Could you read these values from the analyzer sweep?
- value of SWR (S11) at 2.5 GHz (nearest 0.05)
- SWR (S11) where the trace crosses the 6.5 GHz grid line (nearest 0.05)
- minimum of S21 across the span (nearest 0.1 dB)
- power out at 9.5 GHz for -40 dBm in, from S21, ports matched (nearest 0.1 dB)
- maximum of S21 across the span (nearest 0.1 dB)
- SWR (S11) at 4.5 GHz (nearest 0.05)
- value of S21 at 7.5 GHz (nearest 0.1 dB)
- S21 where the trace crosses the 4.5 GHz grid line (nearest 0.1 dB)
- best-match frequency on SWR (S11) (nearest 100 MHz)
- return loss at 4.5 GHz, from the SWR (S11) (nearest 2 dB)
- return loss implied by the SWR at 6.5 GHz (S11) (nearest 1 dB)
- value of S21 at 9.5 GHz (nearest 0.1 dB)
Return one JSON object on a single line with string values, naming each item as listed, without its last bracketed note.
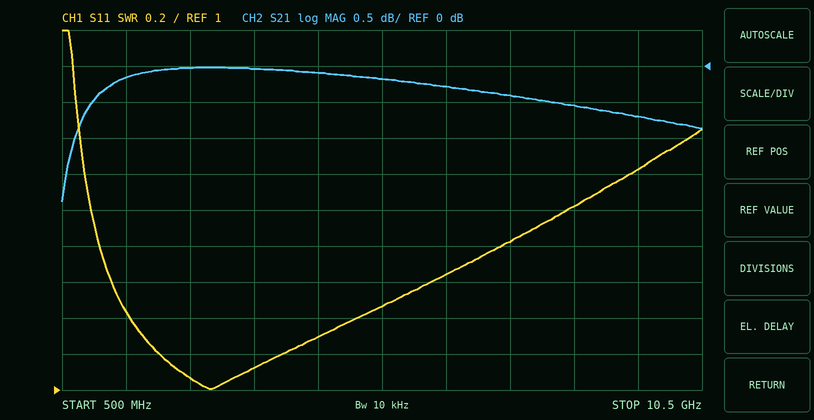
{"value of SWR (S11) at 2.5 GHz": "1.05", "SWR (S11) where the trace crosses the 6.5 GHz grid line": "1.65", "minimum of S21 across the span": "-1.9 dB", "power out at 9.5 GHz for -40 dBm in, from S21, ports matched": "-40.7 dBm", "maximum of S21 across the span": "0.0 dB", "SWR (S11) at 4.5 GHz": "1.30", "value of S21 at 7.5 GHz": "-0.4 dB", "S21 where the trace crosses the 4.5 GHz grid line": "-0.1 dB", "best-match frequency on SWR (S11)": "2.8 GHz", "return loss at 4.5 GHz, from the SWR (S11)": "18 dB", "return loss implied by the SWR at 6.5 GHz (S11)": "12 dB", "value of S21 at 9.5 GHz": "-0.7 dB"}
